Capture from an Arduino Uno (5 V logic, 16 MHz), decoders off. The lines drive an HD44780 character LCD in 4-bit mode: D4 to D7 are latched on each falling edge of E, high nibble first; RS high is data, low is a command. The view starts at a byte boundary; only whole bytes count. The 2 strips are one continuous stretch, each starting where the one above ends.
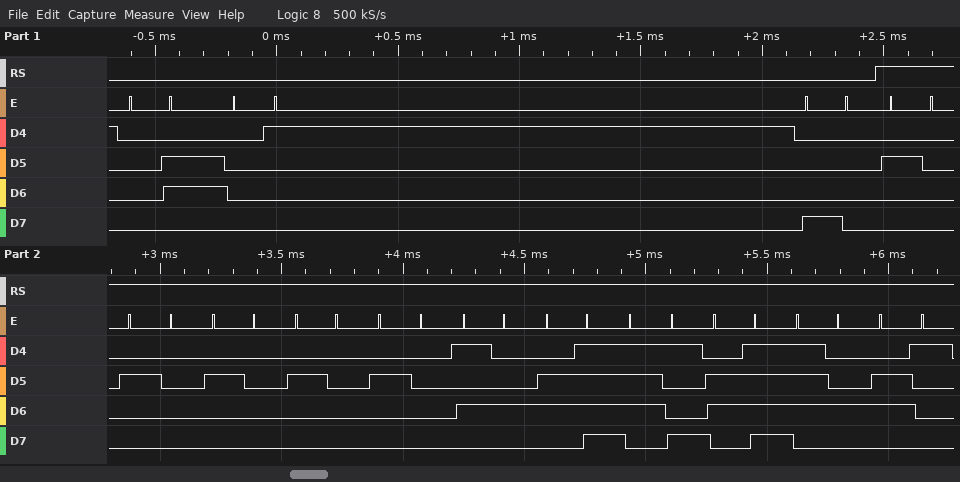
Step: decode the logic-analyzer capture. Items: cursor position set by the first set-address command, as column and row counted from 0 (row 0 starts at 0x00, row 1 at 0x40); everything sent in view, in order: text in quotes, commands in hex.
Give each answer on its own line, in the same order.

column 0, row 0
0x06 0x01 0x80 "     Toyota"
